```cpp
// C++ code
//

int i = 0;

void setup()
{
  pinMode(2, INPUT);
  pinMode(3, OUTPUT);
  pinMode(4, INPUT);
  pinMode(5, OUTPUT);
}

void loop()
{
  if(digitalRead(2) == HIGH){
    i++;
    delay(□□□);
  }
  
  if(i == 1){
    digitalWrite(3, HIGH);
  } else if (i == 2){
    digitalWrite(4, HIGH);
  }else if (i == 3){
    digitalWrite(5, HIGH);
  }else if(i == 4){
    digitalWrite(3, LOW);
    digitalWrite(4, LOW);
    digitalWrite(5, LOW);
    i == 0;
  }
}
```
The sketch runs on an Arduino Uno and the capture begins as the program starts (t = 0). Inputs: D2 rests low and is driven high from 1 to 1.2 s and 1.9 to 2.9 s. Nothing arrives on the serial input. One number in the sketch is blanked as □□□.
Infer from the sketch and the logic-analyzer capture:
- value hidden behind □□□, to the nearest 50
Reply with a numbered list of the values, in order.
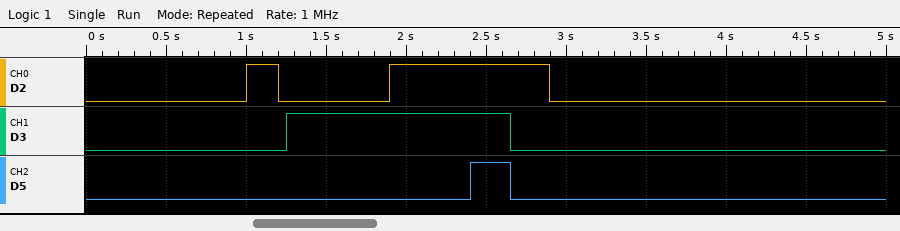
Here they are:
1. 250
